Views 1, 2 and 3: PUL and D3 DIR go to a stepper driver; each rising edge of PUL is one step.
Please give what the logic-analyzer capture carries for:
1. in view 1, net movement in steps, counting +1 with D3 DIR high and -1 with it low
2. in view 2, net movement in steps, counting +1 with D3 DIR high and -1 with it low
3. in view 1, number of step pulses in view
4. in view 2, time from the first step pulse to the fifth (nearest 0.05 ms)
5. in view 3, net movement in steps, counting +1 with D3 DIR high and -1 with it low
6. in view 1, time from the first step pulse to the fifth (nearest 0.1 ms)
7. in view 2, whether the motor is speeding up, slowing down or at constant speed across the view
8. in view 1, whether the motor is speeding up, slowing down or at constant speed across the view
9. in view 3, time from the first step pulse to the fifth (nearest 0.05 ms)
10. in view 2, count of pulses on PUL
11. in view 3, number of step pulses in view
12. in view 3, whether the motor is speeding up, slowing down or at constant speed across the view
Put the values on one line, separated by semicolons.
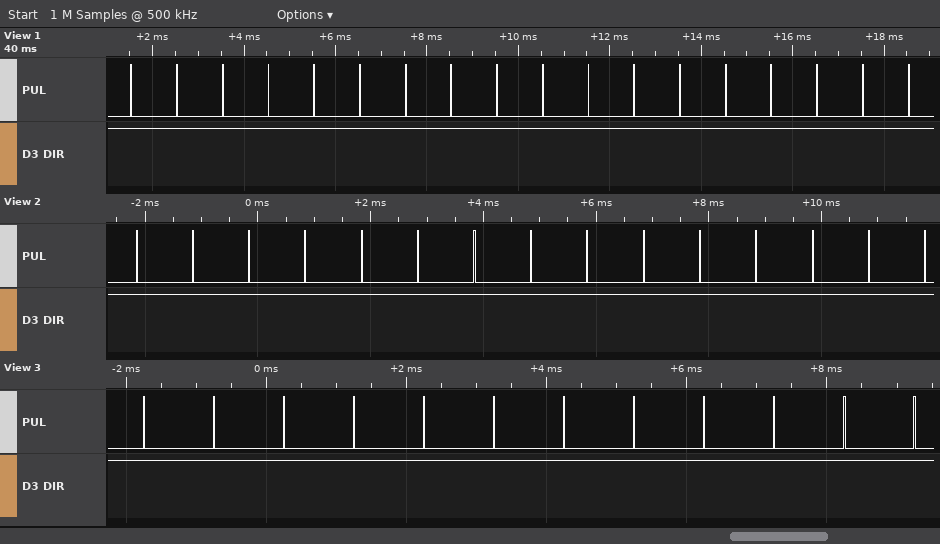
+18; +15; 18; 4.00 ms; +12; 4.0 ms; constant speed; constant speed; 4.00 ms; 15; 12; constant speed
